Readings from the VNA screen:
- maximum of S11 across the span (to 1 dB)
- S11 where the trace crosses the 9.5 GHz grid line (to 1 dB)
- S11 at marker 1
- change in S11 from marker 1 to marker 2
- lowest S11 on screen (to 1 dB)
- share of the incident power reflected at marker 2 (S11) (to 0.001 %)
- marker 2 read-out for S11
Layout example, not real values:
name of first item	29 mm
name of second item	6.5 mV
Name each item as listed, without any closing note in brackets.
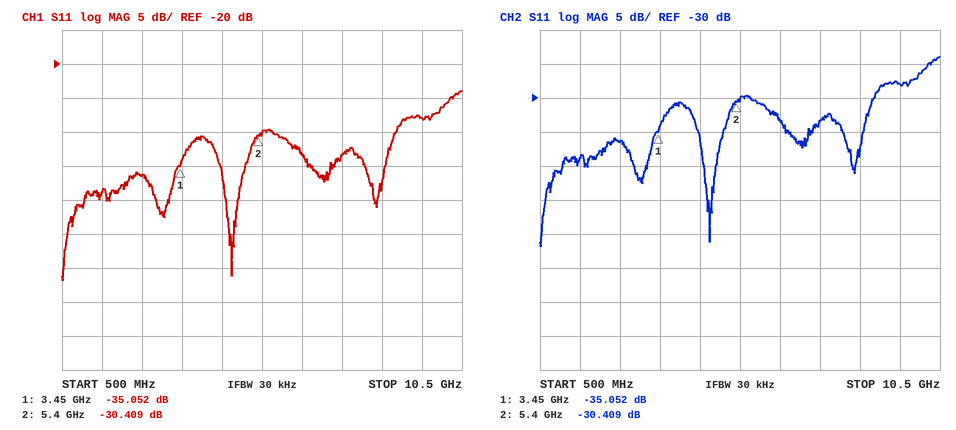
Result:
maximum of S11 across the span	-24 dB
S11 where the trace crosses the 9.5 GHz grid line	-28 dB
S11 at marker 1	-35.052 dB
change in S11 from marker 1 to marker 2	4.643 dB
lowest S11 on screen	-52 dB
share of the incident power reflected at marker 2 (S11)	0.091 %
marker 2 read-out for S11	-30.409 dB
